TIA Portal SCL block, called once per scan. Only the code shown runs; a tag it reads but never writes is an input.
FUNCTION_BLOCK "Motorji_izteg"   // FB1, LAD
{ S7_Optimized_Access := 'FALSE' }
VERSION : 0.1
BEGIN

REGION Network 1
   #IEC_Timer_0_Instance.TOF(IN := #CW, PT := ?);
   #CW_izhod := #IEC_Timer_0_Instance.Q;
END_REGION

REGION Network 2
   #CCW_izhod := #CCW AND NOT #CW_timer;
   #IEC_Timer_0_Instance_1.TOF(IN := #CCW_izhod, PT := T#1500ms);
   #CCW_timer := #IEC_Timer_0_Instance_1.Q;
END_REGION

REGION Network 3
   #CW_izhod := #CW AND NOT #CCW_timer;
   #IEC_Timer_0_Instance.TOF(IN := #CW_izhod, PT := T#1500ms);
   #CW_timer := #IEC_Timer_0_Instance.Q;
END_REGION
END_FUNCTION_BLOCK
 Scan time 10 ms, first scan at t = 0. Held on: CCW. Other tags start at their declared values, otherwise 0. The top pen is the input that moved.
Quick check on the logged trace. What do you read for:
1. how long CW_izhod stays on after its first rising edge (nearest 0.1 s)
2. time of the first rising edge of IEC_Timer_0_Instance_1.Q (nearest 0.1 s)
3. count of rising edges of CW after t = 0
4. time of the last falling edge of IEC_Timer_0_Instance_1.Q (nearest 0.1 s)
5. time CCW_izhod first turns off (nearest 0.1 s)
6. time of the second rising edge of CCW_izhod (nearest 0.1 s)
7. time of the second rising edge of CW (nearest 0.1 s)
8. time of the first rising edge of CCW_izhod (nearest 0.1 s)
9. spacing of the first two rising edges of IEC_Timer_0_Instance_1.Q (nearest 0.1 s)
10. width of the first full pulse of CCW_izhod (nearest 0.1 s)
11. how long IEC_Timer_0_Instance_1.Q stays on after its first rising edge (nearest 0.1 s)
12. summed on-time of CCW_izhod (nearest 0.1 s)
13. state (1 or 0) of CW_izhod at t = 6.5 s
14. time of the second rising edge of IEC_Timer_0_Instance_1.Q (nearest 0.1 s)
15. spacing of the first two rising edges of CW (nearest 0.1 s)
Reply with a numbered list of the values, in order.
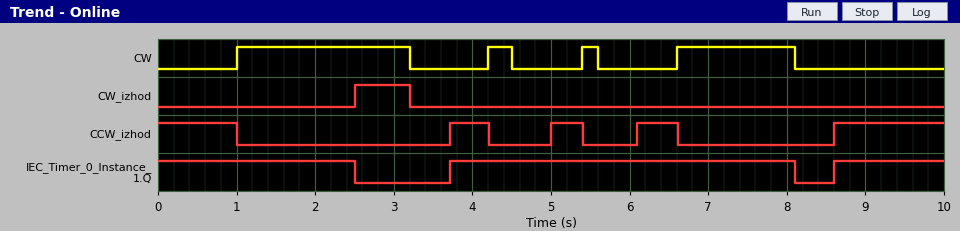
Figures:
1. 0.7 s
2. 3.7 s
3. 4
4. 8.1 s
5. 1.0 s
6. 5.0 s
7. 4.2 s
8. 3.7 s
9. 4.9 s
10. 0.5 s
11. 4.4 s
12. 3.8 s
13. 0
14. 8.6 s
15. 3.2 s
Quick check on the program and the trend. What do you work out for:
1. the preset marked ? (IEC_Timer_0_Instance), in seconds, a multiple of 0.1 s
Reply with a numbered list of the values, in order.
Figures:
1. 0.5 s
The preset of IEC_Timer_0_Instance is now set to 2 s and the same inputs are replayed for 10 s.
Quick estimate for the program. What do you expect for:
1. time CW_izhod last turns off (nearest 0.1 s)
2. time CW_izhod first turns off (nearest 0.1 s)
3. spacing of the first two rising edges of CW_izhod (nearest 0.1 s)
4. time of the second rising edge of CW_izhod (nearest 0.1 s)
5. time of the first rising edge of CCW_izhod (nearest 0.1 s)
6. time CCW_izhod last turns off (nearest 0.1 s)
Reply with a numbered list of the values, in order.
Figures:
1. 8.1 s
2. 3.2 s
3. 1.7 s
4. 4.2 s
5. 9.6 s
6. 1.0 s
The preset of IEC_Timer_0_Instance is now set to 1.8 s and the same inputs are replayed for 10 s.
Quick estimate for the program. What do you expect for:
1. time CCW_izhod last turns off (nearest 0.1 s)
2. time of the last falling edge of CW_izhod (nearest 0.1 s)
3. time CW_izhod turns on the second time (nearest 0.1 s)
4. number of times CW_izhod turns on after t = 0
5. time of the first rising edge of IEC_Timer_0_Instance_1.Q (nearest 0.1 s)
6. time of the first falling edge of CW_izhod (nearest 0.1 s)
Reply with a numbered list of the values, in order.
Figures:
1. 1.0 s
2. 8.1 s
3. 4.2 s
4. 4
5. 9.6 s
6. 3.2 s
